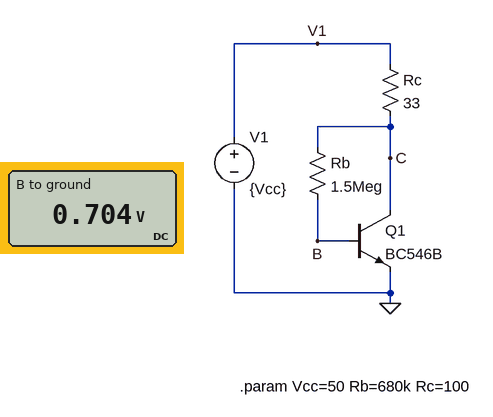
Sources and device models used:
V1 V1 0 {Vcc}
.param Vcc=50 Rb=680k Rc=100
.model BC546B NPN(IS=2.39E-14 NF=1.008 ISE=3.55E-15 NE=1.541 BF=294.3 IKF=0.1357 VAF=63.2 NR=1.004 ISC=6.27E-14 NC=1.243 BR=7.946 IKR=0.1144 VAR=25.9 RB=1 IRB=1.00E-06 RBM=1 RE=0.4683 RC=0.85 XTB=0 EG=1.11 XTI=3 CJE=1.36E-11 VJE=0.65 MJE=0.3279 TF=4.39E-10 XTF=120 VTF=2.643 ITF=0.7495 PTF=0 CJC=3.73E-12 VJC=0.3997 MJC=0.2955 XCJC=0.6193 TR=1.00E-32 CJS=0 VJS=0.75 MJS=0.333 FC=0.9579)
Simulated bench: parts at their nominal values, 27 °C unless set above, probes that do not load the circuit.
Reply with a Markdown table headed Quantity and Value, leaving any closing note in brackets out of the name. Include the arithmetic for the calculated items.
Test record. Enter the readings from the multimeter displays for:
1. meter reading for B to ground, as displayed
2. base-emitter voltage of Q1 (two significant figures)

| Quantity | Value |
|---|---|
| meter reading for B to ground, as displayed | 0.704 V |
| base-emitter voltage of Q1 | 704 mV = 700 mV |
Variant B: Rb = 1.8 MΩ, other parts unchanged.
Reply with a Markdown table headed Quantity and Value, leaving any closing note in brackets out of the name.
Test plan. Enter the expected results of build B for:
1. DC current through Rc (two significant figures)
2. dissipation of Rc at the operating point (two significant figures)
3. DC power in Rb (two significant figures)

| Quantity | Value |
|---|---|
| DC current through Rc | 13 mA |
| dissipation of Rc at the operating point | 5.7 mW |
| DC power in Rb | 1.3 mW |
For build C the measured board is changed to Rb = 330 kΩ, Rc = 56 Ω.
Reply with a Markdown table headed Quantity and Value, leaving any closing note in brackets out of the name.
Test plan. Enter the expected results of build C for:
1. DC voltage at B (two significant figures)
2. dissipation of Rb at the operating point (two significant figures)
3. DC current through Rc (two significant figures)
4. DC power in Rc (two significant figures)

| Quantity | Value |
|---|---|
| DC voltage at B | 760 mV |
| dissipation of Rb at the operating point | 6.4 mW |
| DC current through Rc | 56 mA |
| DC power in Rc | 180 mW |
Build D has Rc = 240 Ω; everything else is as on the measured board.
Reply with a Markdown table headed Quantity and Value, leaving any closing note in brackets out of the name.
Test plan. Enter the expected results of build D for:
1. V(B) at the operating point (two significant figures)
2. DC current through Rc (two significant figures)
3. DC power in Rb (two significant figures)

| Quantity | Value |
|---|---|
| V(B) at the operating point | 700 mV |
| DC current through Rc | 14 mA |
| DC power in Rb | 1.4 mW |
